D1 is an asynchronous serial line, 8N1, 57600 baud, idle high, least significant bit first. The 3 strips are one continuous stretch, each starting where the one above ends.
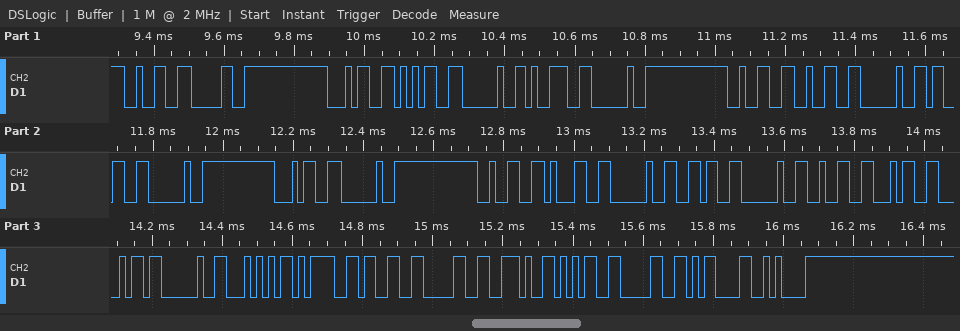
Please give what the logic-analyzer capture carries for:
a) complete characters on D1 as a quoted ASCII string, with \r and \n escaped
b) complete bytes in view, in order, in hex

"2045 9 22 3 4 21 6 24h T=30.50\r\n"
0x32 0x30 0x34 0x35 0x20 0x39 0x20 0x32 0x32 0x20 0x33 0x20 0x34 0x20 0x32 0x31 0x20 0x36 0x20 0x32 0x34 0x68 0x20 0x54 0x3D 0x33 0x30 0x2E 0x35 0x30 0x0D 0x0A
